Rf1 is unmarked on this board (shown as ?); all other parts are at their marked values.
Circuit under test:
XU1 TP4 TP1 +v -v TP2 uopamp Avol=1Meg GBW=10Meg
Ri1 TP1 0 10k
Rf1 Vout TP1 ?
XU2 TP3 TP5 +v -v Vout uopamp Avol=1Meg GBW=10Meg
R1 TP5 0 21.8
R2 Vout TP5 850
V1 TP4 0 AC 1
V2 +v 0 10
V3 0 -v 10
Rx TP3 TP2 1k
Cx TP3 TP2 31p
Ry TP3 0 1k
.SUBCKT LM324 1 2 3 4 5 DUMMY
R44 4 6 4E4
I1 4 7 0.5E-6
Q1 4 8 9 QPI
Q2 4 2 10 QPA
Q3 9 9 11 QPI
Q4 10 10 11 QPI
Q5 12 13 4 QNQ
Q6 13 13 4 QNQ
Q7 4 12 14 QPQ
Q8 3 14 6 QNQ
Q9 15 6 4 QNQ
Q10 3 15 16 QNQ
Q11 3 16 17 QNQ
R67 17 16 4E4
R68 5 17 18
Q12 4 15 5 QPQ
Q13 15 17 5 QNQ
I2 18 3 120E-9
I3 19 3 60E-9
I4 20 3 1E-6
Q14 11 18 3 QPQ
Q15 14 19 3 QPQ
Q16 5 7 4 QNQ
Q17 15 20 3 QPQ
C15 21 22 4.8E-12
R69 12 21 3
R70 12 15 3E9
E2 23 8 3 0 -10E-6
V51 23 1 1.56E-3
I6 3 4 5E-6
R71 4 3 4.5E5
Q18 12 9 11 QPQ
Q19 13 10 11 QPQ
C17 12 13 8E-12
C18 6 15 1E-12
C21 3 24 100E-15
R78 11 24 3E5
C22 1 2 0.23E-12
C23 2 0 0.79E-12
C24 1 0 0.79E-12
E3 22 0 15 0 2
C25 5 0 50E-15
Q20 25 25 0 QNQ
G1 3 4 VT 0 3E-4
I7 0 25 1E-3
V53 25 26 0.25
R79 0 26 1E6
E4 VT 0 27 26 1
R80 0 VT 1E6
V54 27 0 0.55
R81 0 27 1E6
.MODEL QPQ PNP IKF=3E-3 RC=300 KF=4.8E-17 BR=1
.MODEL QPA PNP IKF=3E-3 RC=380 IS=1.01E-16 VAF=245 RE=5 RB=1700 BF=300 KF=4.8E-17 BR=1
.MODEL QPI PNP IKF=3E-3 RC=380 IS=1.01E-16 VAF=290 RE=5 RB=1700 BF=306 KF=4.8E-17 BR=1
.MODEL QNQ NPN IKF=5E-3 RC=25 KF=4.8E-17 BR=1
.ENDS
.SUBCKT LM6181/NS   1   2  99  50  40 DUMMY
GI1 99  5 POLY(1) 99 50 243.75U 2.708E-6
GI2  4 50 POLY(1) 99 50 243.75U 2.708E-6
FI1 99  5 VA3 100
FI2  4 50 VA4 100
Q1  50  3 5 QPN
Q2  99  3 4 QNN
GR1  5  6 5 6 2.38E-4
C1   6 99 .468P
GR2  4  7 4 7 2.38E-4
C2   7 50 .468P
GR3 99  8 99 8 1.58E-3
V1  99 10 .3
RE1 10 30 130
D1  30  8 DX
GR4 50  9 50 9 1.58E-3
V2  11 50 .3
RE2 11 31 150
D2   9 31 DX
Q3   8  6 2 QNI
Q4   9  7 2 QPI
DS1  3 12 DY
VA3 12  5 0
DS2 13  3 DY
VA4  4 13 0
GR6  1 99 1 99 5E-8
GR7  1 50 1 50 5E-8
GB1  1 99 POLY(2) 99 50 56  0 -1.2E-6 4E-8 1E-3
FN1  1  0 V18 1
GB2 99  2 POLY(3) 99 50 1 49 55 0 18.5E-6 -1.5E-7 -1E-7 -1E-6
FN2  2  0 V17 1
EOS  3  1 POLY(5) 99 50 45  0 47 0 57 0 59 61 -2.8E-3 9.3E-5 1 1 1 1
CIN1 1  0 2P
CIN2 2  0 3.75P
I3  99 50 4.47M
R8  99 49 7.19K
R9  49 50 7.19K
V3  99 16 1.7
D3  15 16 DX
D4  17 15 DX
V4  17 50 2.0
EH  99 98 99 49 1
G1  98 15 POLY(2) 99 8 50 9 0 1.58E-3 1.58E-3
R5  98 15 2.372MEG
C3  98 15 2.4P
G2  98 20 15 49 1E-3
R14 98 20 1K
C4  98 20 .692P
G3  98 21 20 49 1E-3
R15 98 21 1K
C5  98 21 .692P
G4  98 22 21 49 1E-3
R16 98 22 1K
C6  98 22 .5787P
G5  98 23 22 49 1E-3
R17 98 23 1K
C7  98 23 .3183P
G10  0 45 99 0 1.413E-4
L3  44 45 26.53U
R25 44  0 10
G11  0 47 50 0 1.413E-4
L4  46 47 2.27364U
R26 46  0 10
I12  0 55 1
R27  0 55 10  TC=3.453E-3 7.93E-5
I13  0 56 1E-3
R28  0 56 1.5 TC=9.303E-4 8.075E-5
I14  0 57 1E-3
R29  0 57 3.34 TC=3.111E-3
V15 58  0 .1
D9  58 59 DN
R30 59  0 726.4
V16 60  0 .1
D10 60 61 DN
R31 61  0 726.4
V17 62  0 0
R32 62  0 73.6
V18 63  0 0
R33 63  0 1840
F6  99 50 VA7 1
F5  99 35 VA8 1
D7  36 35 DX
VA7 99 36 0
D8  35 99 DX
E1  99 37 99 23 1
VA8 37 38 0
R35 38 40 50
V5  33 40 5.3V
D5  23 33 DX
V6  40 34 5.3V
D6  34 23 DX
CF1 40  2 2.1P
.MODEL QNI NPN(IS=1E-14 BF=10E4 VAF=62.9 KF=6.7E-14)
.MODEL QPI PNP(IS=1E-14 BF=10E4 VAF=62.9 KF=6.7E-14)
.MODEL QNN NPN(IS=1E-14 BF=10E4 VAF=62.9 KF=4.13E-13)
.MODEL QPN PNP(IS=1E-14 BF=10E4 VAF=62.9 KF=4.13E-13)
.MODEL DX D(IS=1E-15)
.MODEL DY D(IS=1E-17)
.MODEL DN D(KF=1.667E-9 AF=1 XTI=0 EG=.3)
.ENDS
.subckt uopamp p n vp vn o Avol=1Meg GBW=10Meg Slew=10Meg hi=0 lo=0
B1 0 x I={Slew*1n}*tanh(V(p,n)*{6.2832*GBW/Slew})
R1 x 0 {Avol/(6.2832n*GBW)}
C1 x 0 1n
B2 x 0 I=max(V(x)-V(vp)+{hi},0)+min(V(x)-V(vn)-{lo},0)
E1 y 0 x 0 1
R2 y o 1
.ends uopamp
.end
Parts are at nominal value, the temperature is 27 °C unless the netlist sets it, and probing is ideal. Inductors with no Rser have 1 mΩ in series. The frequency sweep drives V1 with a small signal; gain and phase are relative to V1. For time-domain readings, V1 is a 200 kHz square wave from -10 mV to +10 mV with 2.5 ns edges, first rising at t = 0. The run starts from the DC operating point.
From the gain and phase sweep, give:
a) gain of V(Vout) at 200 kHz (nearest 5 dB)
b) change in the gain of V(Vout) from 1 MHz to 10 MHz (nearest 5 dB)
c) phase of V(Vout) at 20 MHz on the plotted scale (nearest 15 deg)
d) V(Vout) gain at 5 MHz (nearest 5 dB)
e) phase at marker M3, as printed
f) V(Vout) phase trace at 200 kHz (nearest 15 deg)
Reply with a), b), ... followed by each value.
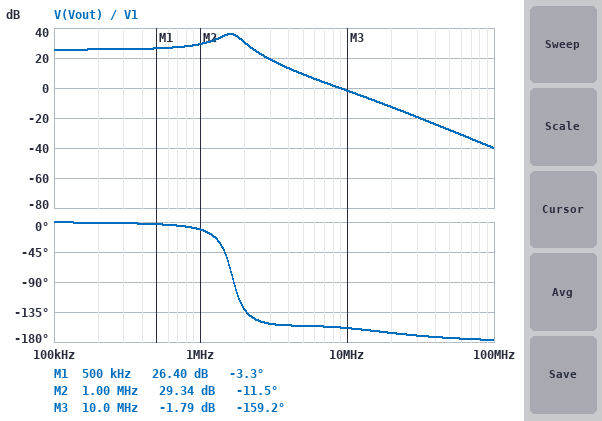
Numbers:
a) 25 dB
b) -30 dB
c) -165 deg
d) 10 dB
e) -159.2 deg
f) 0 deg
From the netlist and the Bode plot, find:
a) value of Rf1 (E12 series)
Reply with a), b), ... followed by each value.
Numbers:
a) 180 kΩ
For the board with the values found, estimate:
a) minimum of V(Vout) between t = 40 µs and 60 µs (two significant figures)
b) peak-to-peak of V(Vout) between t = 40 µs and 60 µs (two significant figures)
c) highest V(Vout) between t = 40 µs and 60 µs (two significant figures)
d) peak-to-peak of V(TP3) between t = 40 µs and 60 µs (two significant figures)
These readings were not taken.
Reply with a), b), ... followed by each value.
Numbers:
a) -430 mV
b) 860 mV
c) 430 mV
d) 110 mV
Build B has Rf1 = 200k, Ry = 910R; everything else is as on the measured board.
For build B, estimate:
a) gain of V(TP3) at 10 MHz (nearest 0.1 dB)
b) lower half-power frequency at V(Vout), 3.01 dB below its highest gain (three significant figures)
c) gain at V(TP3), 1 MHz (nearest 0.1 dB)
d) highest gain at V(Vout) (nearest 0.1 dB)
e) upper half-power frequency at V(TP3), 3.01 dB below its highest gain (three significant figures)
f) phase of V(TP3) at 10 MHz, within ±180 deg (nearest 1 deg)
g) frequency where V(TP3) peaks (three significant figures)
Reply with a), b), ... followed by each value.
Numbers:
a) -2.0 dB
b) 1.22 MHz
c) 11.2 dB
d) 36.7 dB
e) 1.79 MHz
f) -69 deg
g) 1.52 MHz
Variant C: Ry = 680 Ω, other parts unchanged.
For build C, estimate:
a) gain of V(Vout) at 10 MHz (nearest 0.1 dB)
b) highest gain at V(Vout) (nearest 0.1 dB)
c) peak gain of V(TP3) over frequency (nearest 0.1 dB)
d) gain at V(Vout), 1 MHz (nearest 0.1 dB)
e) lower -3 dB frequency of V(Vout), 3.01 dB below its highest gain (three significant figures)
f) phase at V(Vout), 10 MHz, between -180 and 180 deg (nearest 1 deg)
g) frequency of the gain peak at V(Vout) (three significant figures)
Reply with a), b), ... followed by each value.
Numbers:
a) -2.9 dB
b) 35.3 dB
c) 18.7 dB
d) 30.3 dB
e) 1.15 MHz
f) -153 deg
g) 1.43 MHz
